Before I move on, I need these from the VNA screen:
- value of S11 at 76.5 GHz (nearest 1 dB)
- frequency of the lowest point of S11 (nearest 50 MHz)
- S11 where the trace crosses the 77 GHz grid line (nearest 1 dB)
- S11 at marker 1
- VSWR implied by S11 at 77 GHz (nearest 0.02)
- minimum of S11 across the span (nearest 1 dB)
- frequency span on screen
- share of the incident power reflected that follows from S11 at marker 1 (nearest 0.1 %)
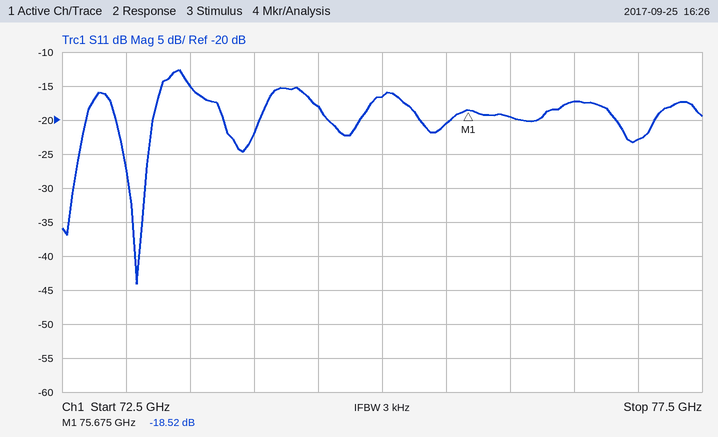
-17 dB
73.10 GHz
-23 dB
-18.52 dB
1.16
-44 dB
5 GHz
1.4 %
